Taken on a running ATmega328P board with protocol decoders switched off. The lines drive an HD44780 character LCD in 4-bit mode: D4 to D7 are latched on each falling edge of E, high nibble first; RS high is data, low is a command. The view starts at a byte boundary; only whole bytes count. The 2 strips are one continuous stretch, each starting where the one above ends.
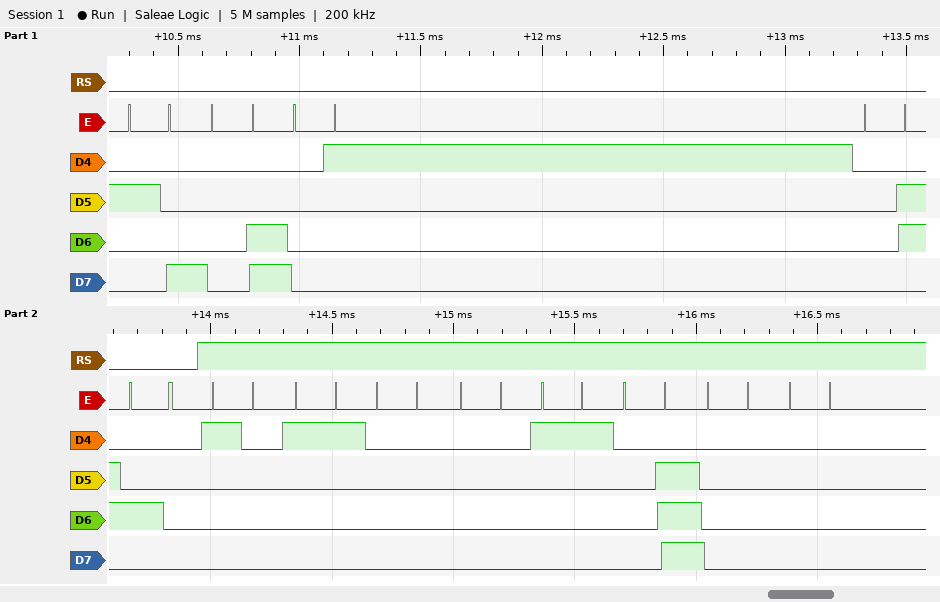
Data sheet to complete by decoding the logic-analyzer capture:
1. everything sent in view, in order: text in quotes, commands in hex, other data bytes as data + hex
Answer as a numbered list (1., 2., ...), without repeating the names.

1. 0x28 0x0C 0x01 0x06 0x40 data 10 11 00 00 11 0E 00 00
